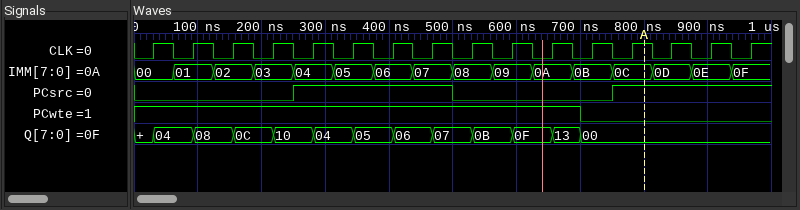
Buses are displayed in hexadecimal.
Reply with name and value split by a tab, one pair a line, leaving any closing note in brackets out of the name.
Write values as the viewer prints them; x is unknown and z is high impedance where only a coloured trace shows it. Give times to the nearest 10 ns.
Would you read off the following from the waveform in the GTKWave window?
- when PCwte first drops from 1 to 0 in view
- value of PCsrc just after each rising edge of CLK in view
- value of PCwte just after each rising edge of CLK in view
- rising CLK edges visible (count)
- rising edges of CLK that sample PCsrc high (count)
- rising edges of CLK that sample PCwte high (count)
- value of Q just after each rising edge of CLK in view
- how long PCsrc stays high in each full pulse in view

when PCwte first drops from 1 to 0 in view	700 ns
value of PCsrc just after each rising edge of CLK in view	0 0 0 0 1 1 1 1 0 0 0 0 1 1 1 1
value of PCwte just after each rising edge of CLK in view	1 1 1 1 1 1 1 1 1 1 1 0 0 0 0 0
rising CLK edges visible	16
rising edges of CLK that sample PCsrc high	8
rising edges of CLK that sample PCwte high	11
value of Q just after each rising edge of CLK in view	04, 08, 0C, 10, 04, 05, 06, 07, 0B, 0F, 13, 00, 00, 00, 00, 00
how long PCsrc stays high in each full pulse in view	250 ns
